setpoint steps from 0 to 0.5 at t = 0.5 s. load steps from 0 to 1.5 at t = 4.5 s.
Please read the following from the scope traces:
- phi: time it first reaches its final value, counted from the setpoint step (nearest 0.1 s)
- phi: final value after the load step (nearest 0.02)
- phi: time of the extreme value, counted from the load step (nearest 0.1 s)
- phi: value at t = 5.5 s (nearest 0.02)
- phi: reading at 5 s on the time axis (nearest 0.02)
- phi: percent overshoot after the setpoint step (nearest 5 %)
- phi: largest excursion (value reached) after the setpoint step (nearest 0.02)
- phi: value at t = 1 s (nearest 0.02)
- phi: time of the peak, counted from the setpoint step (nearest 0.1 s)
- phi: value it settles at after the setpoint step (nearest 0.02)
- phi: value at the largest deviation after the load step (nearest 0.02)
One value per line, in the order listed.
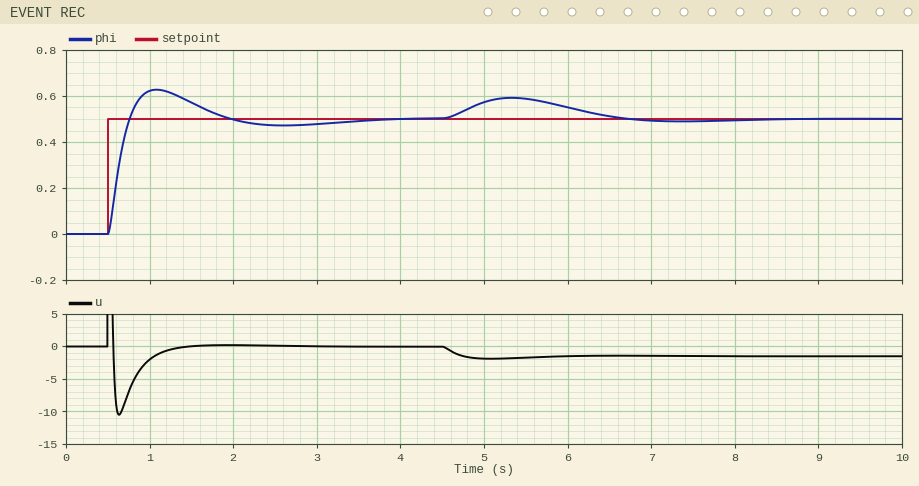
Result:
0.3 s
0.50
0.8 s
0.58
0.58
25 %
0.62
0.62
0.6 s
0.50
0.60
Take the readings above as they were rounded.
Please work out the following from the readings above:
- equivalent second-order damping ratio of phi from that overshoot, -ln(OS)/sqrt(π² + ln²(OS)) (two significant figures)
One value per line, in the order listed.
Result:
0.40
